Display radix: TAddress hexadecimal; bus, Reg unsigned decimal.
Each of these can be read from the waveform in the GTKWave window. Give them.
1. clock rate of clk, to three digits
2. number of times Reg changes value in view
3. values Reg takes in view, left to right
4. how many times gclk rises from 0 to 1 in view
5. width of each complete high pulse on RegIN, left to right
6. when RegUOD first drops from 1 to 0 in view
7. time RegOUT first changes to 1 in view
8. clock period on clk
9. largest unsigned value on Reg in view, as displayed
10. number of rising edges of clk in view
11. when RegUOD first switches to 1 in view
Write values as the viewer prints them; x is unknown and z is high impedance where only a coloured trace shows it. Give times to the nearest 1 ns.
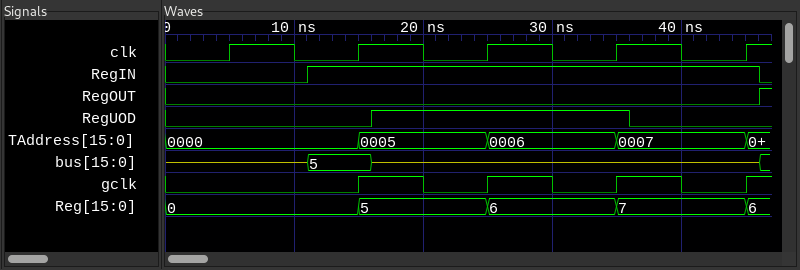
100 MHz
4
0, 5, 6, 7, 6
4
35 ns
36 ns
46 ns
10 ns
7
5
16 ns
